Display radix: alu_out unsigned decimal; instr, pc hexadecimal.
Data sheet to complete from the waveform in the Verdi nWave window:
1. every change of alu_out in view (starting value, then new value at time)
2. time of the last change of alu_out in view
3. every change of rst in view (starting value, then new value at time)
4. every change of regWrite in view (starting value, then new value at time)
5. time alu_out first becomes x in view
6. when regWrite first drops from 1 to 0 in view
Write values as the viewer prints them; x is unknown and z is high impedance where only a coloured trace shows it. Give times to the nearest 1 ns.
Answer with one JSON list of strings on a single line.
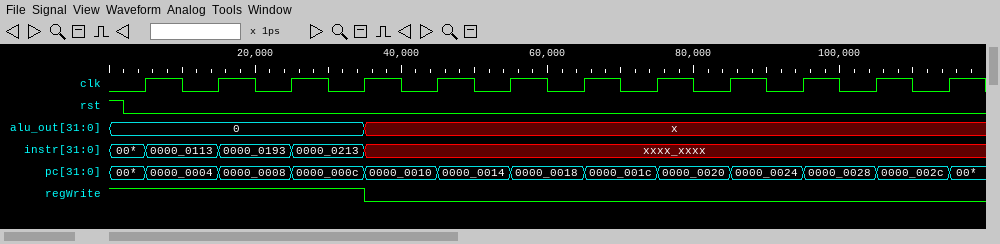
["0, x at 35 ns", "35 ns", "1, 0 at 2 ns", "1, 0 at 35 ns", "35 ns", "35 ns"]
